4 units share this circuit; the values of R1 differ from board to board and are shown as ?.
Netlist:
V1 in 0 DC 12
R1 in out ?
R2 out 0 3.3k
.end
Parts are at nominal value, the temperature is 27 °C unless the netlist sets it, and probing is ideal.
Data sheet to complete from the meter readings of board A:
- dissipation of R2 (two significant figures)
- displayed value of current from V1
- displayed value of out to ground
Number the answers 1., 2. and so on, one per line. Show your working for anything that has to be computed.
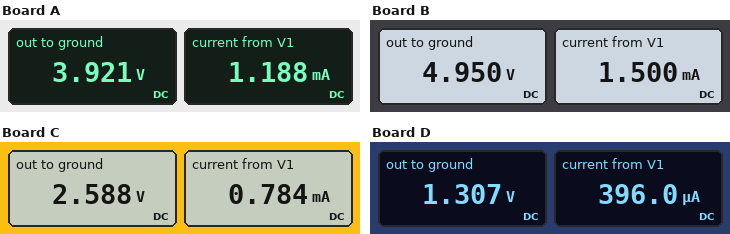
1. (3.921 V)^2 / 3.3 kΩ = 4.7 mW
2. 1.188 mA
3. 3.921 V
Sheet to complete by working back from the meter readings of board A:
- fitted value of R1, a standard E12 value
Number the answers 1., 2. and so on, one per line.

1. 6.8 kΩ
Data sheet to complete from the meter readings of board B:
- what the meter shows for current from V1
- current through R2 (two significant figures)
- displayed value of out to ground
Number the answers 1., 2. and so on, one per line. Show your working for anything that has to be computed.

1. 1.500 mA
2. (4.95 V) / 3.3 kΩ = 1.5 mA
3. 4.950 V
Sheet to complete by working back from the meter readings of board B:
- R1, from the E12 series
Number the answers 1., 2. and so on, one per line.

1. 4.7 kΩ
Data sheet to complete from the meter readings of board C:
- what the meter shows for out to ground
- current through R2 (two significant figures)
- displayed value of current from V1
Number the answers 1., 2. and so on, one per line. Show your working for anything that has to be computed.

1. 2.588 V
2. (2.588 V) / 3.3 kΩ = 780 µA
3. 0.784 mA
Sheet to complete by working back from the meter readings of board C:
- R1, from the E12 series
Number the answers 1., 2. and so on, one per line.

1. 12 kΩ
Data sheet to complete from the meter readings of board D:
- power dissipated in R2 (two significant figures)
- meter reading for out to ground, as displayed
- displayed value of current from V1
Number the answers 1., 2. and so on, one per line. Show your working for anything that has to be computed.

1. (1.307 V)^2 / 3.3 kΩ = 520 µW
2. 1.307 V
3. 396.0 µA
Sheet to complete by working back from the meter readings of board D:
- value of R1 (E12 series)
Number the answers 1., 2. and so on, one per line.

1. 27 kΩ
